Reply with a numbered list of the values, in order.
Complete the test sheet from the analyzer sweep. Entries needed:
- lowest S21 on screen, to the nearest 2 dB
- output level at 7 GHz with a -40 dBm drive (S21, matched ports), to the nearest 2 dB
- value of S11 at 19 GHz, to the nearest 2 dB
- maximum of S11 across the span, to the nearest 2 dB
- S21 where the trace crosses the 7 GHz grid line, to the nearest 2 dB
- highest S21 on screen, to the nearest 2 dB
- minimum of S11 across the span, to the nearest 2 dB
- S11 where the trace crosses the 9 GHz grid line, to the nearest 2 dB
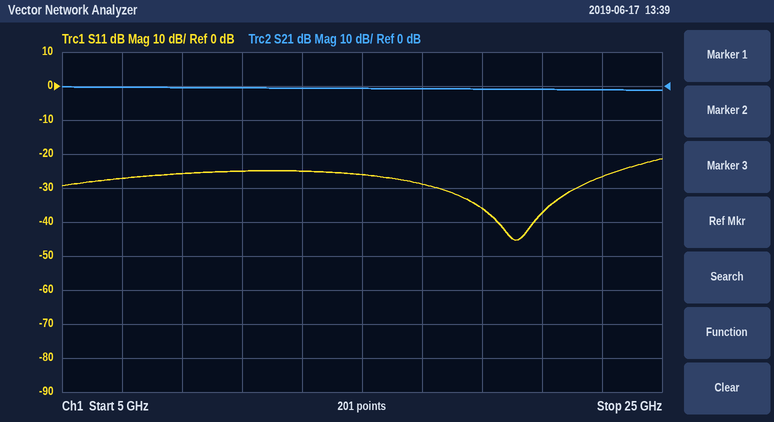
1. -2 dB
2. -40 dBm
3. -36 dB
4. -22 dB
5. 0 dB
6. 0 dB
7. -46 dB
8. -26 dB
